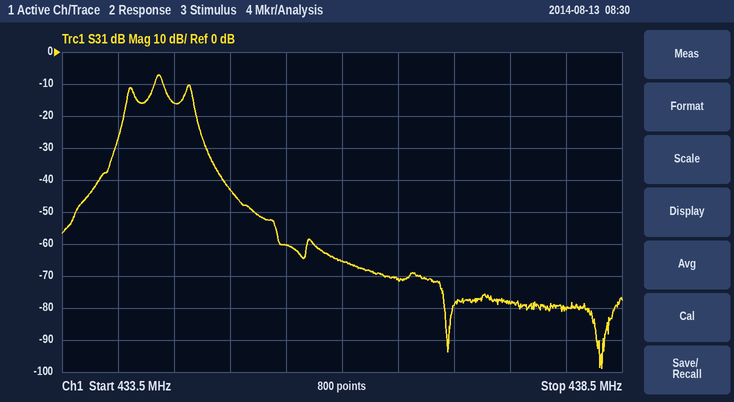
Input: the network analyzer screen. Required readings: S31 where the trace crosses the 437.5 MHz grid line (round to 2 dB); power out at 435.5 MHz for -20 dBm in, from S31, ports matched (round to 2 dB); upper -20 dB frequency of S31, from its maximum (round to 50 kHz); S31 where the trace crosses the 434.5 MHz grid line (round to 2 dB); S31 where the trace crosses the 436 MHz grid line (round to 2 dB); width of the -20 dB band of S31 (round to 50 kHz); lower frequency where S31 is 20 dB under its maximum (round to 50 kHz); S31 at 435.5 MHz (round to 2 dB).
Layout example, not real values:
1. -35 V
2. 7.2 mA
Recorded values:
1. -78 dB
2. -80 dBm
3. 434.75 MHz
4. -16 dB
5. -66 dB
6. 750 kHz
7. 434.00 MHz
8. -60 dB
